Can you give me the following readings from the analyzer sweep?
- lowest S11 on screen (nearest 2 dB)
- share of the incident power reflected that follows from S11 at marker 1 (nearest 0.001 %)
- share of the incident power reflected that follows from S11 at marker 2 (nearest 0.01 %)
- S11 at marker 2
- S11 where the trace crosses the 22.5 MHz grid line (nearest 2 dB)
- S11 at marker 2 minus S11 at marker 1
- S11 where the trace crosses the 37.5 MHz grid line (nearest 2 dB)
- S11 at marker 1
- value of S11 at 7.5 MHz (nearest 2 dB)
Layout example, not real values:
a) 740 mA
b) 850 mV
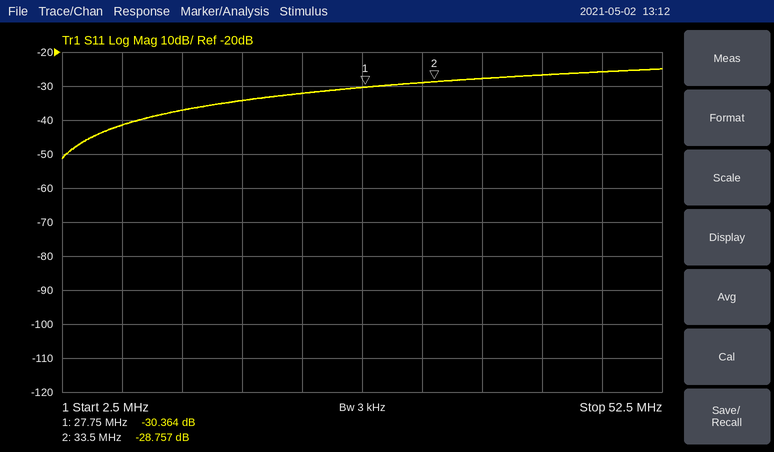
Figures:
a) -52 dB
b) 0.092 %
c) 0.13 %
d) -28.757 dB
e) -32 dB
f) 1.607 dB
g) -28 dB
h) -30.364 dB
i) -42 dB
